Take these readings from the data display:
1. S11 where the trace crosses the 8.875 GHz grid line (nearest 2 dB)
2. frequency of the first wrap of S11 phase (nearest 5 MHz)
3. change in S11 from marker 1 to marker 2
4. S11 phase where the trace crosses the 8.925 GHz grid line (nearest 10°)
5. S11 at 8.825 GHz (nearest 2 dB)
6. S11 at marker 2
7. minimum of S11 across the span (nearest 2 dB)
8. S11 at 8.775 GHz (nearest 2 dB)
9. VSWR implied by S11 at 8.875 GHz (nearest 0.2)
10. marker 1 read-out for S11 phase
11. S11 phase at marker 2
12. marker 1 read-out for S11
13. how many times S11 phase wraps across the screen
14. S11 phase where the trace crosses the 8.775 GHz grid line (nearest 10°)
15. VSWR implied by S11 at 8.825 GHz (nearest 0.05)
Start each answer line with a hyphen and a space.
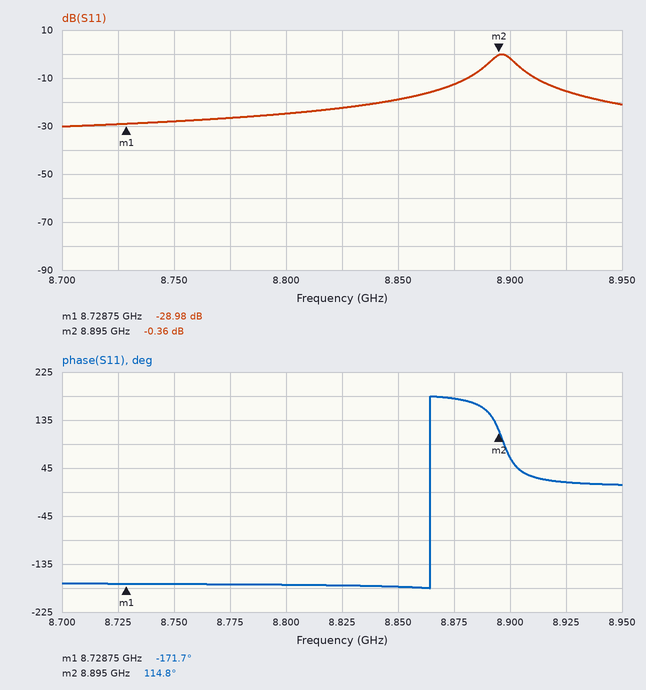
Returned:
- -12 dB
- 8.865 GHz
- 28.62 dB
- 20°
- -22 dB
- -0.36 dB
- -30 dB
- -26 dB
- 1.6
- -171.7°
- 114.8°
- -28.98 dB
- 1
- -170°
- 1.15
